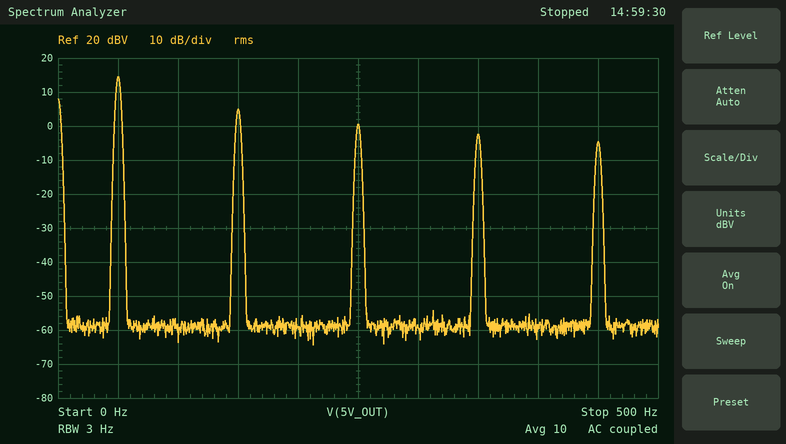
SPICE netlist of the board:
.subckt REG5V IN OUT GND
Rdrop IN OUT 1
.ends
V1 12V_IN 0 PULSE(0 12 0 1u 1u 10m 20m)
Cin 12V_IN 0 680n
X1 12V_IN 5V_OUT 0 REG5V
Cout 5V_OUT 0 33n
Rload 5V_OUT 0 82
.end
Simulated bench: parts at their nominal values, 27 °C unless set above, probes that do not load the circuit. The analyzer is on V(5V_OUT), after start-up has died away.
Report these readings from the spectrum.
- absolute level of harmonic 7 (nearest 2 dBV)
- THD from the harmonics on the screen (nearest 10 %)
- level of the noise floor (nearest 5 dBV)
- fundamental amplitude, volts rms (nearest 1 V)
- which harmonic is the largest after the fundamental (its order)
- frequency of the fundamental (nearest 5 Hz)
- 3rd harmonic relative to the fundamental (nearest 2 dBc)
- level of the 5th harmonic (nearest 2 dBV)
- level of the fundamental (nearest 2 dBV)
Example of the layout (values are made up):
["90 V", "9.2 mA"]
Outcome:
["-2 dBV", "40 %", "-60 dBV", "5 V", "3", "50 Hz", "-10 dBc", "0 dBV", "14 dBV"]
